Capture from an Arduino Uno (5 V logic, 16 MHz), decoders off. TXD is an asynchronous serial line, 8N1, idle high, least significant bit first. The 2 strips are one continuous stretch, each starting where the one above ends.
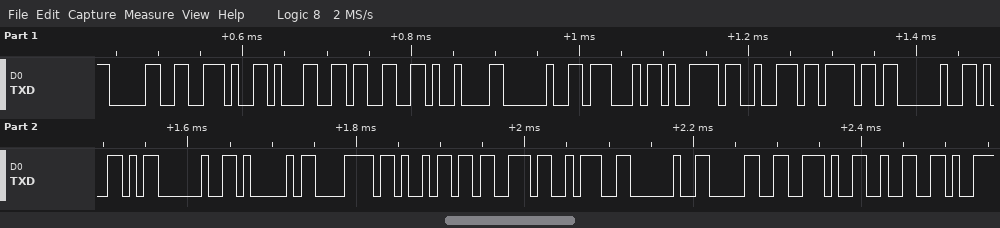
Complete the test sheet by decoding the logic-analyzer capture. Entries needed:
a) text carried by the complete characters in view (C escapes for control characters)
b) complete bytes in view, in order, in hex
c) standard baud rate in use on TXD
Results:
"0.13\t Gyro Y Axis: 0.2"
30 2E 31 33 09 20 47 79 72 6F 20 59 20 41 78 69 73 3A 20 30 2E 32
115200 baud
